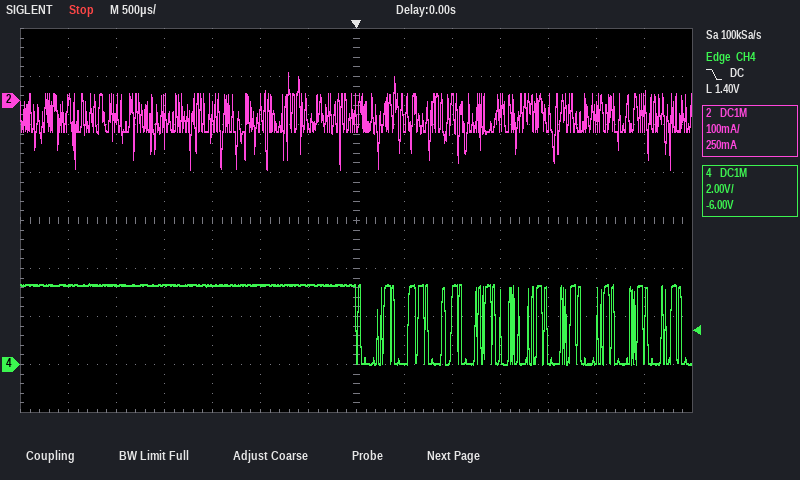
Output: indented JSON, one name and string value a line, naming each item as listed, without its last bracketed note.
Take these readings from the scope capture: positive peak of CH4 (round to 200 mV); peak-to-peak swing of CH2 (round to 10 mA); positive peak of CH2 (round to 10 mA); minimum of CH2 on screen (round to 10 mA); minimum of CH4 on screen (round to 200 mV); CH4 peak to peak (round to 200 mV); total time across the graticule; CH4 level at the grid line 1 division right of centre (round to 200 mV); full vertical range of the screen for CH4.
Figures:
{
  "positive peak of CH4": "3.4 V",
  "peak-to-peak swing of CH2": "200 mA",
  "positive peak of CH2": "60 mA",
  "minimum of CH2 on screen": "-140 mA",
  "minimum of CH4 on screen": "0.0 V",
  "CH4 peak to peak": "3.4 V",
  "total time across the graticule": "7 ms",
  "CH4 level at the grid line 1 division right of centre": "0.0 V",
  "full vertical range of the screen for CH4": "16 V"
}
